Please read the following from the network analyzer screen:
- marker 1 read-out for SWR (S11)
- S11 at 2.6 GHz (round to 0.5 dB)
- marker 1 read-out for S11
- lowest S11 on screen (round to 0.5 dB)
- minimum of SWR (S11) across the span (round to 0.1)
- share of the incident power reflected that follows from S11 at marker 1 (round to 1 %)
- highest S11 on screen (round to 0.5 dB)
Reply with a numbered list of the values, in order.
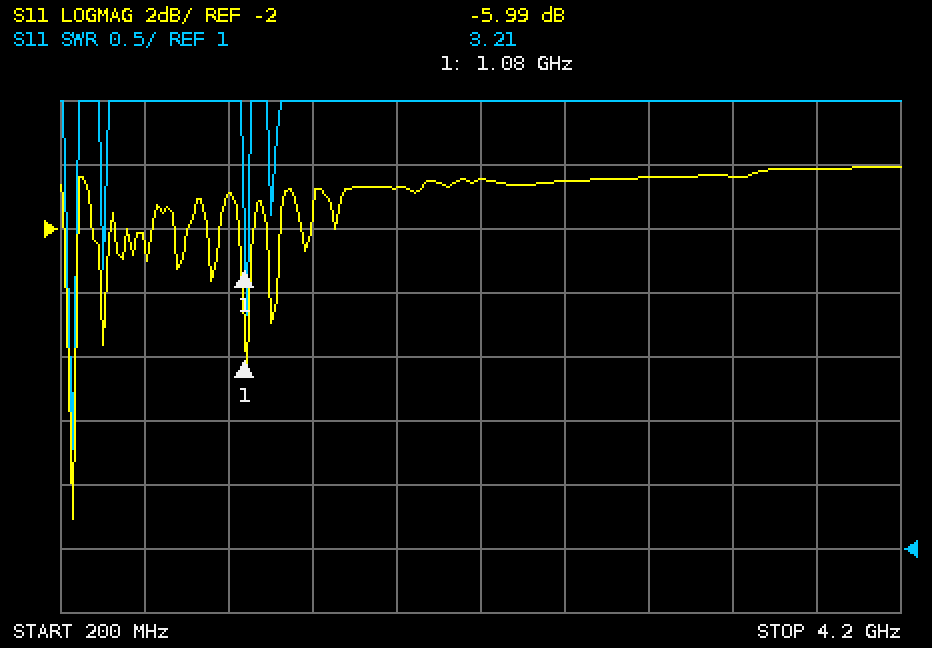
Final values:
1. 3.21
2. -0.5 dB
3. -5.99 dB
4. -11.0 dB
5. 1.8
6. 25 %
7. 0.0 dB
